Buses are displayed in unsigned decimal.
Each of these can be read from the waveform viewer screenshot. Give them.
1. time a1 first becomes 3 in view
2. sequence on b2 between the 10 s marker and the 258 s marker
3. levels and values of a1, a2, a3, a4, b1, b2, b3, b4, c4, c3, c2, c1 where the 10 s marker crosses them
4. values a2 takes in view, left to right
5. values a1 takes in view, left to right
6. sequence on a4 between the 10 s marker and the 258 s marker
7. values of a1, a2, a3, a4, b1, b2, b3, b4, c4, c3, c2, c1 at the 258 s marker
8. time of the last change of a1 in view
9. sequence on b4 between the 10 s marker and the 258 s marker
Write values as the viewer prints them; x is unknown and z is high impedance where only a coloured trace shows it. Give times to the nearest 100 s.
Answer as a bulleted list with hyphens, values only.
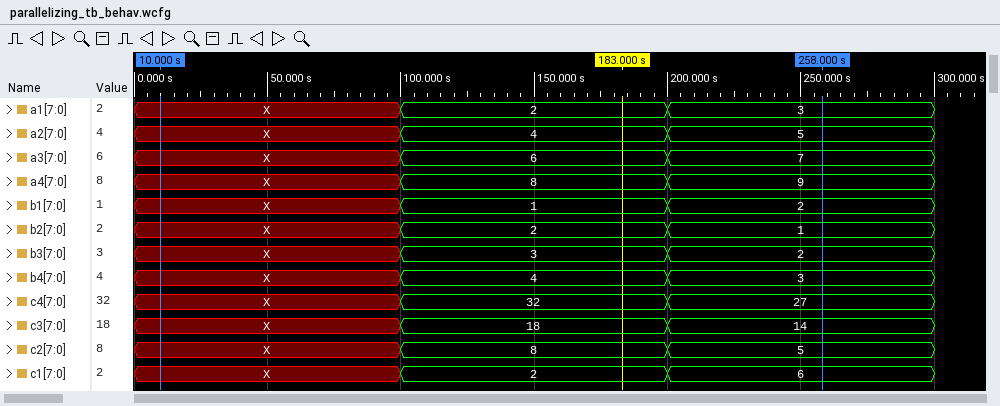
- 200 s
- X, 2, 1
- a1=X, a2=X, a3=X, a4=X, b1=X, b2=X, b3=X, b4=X, c4=X, c3=X, c2=X, c1=X
- X, 4, 5
- X, 2, 3
- X, 8, 9
- a1=3, a2=5, a3=7, a4=9, b1=2, b2=1, b3=2, b4=3, c4=27, c3=14, c2=5, c1=6
- 200 s
- X, 4, 3
